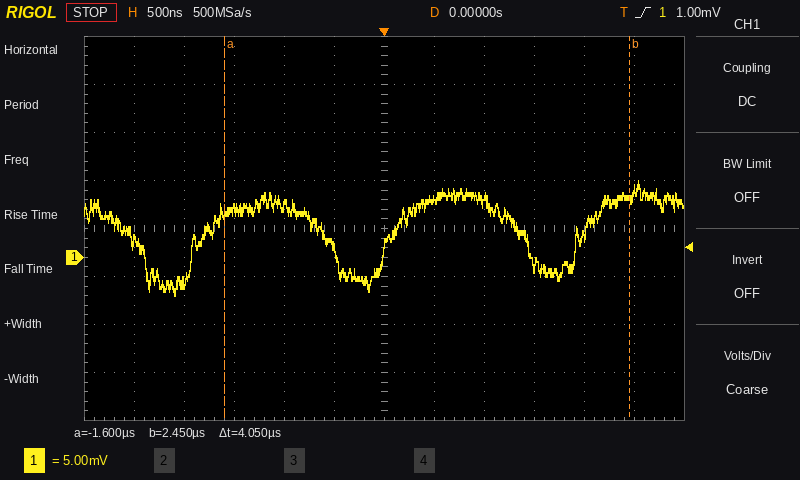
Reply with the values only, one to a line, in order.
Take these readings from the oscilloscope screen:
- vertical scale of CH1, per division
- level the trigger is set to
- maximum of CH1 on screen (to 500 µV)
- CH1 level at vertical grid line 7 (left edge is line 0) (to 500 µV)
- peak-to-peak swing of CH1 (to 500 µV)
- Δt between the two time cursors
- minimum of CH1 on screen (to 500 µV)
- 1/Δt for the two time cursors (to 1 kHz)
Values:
5 mV
1.00 mV
8.0 mV
6.0 mV
12.0 mV
4.05 µs
-4.0 mV
247 kHz
